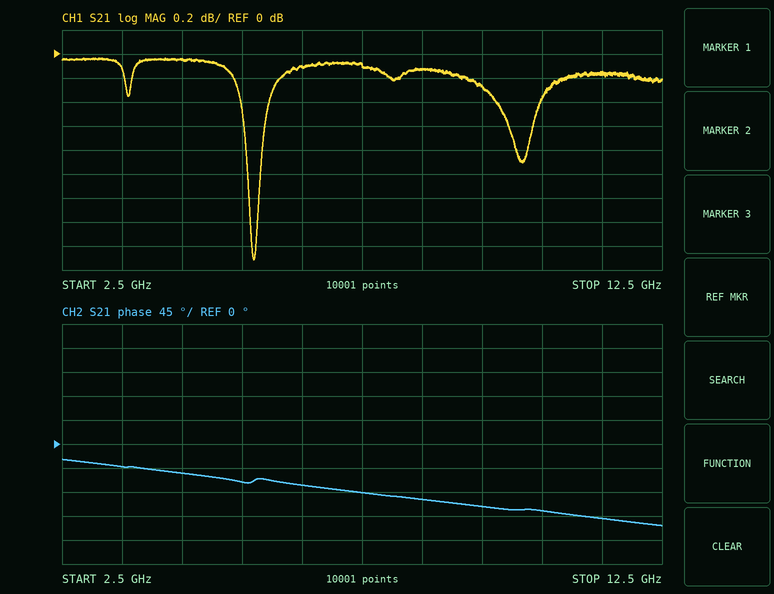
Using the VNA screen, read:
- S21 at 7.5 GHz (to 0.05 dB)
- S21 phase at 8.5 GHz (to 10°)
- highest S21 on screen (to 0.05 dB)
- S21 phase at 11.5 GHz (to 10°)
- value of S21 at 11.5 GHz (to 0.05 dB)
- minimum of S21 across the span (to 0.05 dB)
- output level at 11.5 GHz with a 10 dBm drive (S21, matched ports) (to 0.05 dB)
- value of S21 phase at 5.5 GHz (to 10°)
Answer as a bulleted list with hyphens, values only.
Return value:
- -0.10 dB
- -100°
- -0.05 dB
- -140°
- -0.15 dB
- -1.70 dB
- 9.85 dBm
- -70°
